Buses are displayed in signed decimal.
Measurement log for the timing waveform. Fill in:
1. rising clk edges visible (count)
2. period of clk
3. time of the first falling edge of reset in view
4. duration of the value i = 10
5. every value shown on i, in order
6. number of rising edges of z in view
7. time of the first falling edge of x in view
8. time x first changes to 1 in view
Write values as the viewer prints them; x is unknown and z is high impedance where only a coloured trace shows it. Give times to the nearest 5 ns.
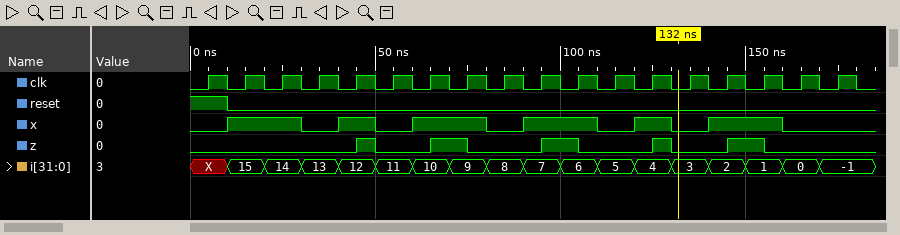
18
10 ns
10 ns
10 ns
X, 15, 14, 13, 12, 11, 10, 9, 8, 7, 6, 5, 4, 3, 2, 1, 0, -1
5
30 ns
10 ns
